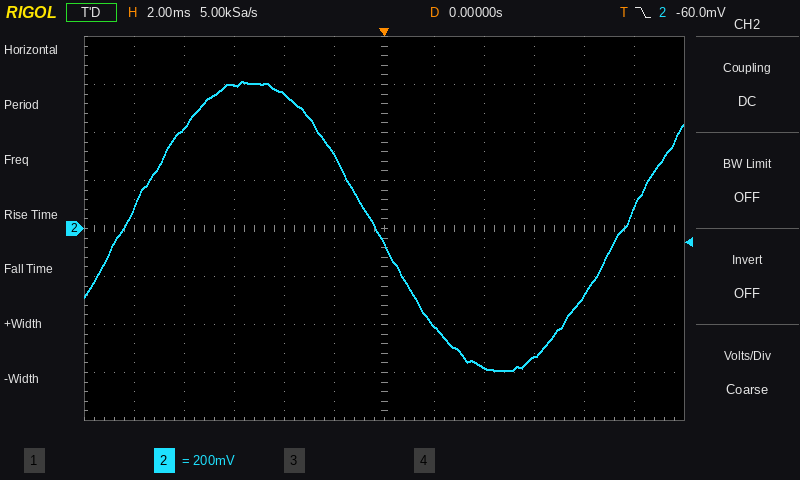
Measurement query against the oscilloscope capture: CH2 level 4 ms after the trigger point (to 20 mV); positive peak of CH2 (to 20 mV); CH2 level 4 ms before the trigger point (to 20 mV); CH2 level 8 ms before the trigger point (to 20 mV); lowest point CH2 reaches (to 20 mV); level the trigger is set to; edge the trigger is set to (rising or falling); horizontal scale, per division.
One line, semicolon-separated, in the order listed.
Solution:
-580 mV; 620 mV; 560 mV; 420 mV; -600 mV; -60.0 mV; falling; 2 ms
